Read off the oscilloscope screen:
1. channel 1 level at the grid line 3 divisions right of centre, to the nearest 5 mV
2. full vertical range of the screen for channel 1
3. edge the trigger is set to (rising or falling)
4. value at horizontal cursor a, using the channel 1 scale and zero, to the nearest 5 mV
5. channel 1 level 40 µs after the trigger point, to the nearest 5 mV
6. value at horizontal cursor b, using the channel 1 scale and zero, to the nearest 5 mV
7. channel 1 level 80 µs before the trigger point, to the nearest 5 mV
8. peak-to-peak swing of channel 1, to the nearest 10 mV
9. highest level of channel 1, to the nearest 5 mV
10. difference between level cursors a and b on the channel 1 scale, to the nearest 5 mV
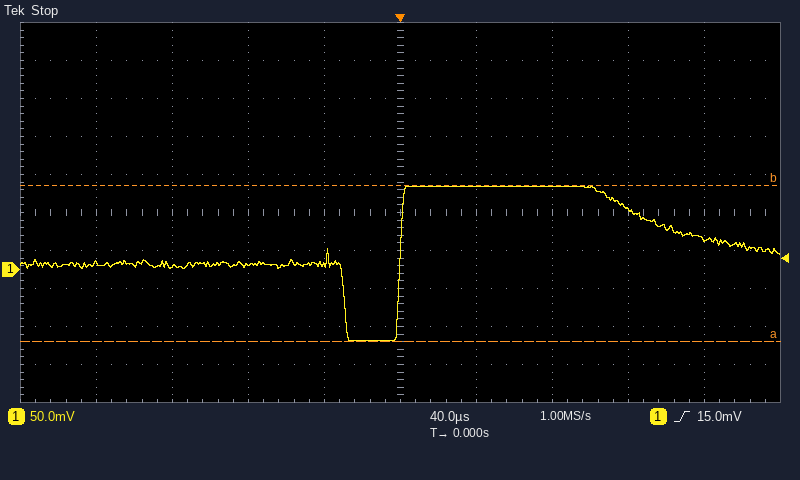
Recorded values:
80 mV
500 mV
rising
-95 mV
110 mV
110 mV
5 mV
200 mV
110 mV
205 mV
